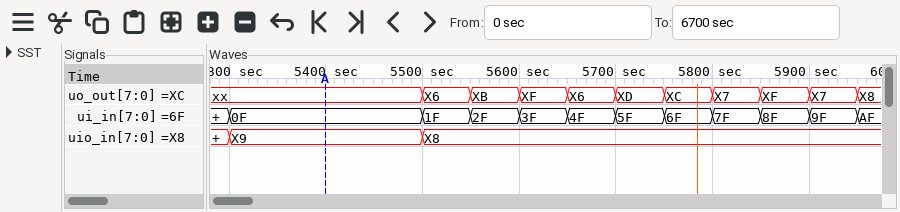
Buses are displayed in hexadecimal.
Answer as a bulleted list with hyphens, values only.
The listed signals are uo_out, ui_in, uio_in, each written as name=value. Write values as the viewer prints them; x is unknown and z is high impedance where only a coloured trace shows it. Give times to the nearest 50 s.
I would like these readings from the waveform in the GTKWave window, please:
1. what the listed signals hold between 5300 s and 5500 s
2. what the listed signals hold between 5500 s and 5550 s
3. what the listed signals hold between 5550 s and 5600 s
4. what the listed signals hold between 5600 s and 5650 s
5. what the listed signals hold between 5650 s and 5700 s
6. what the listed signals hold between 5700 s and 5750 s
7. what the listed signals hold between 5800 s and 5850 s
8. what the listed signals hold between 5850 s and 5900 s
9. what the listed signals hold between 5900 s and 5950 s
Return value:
- uo_out=xx, ui_in=0F, uio_in=X9
- uo_out=X6, ui_in=1F, uio_in=X8
- uo_out=XB, ui_in=2F, uio_in=X8
- uo_out=XF, ui_in=3F, uio_in=X8
- uo_out=X6, ui_in=4F, uio_in=X8
- uo_out=XD, ui_in=5F, uio_in=X8
- uo_out=X7, ui_in=7F, uio_in=X8
- uo_out=XF, ui_in=8F, uio_in=X8
- uo_out=X7, ui_in=9F, uio_in=X8
